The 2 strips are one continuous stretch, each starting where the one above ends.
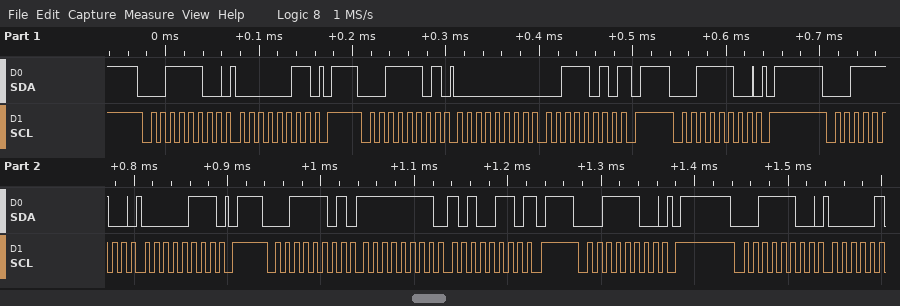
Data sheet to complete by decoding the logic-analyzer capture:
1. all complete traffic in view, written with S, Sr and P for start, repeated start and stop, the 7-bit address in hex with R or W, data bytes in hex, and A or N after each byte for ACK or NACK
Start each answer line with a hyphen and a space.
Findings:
- S 1EW A 03 A P S 1ER A 00 A 3A N P S 1EW A P S 1EW A 07 A P S 1ER A FF A A6 N P S 1EW A P S 1EW A
